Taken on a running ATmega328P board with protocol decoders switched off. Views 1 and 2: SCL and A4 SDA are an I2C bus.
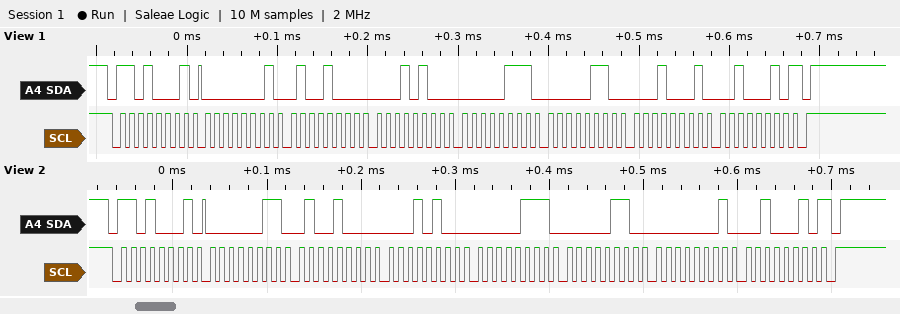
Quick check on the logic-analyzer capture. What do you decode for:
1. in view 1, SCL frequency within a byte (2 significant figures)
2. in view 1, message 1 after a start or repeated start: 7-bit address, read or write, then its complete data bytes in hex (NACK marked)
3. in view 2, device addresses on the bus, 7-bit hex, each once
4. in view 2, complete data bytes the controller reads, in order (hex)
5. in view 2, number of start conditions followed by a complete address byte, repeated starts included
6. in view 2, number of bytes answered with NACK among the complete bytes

100 kHz
0x68 read: 01 48 14 07 06 11 22 NACK
0x68
03 48 14 07 06 01 22
1
1
